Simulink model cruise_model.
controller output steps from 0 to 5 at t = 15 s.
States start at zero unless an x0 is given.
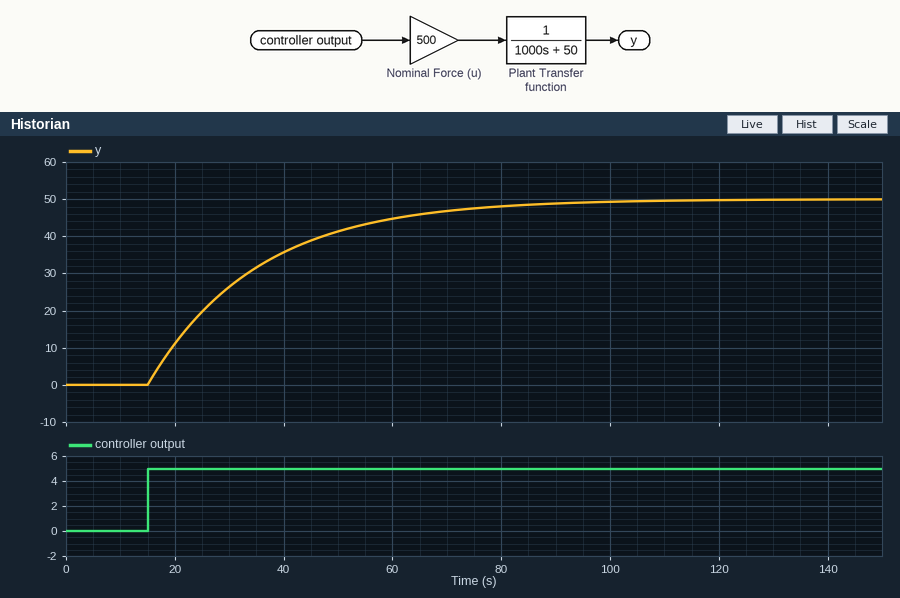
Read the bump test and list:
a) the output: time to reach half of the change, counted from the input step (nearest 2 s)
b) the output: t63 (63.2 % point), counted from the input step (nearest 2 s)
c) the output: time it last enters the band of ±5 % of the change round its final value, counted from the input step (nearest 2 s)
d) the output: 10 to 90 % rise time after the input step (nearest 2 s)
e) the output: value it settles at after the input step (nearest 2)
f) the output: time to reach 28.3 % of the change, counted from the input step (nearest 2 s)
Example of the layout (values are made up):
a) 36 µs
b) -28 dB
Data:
a) 14 s
b) 20 s
c) 60 s
d) 44 s
e) 50
f) 6 s
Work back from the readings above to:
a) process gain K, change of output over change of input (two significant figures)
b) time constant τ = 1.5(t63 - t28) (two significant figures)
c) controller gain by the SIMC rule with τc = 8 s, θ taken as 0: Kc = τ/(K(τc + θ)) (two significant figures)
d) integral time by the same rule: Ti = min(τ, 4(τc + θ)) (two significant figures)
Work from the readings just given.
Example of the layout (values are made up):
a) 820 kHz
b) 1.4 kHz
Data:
a) 10
b) 21 s
c) 0.26
d) 21 s
